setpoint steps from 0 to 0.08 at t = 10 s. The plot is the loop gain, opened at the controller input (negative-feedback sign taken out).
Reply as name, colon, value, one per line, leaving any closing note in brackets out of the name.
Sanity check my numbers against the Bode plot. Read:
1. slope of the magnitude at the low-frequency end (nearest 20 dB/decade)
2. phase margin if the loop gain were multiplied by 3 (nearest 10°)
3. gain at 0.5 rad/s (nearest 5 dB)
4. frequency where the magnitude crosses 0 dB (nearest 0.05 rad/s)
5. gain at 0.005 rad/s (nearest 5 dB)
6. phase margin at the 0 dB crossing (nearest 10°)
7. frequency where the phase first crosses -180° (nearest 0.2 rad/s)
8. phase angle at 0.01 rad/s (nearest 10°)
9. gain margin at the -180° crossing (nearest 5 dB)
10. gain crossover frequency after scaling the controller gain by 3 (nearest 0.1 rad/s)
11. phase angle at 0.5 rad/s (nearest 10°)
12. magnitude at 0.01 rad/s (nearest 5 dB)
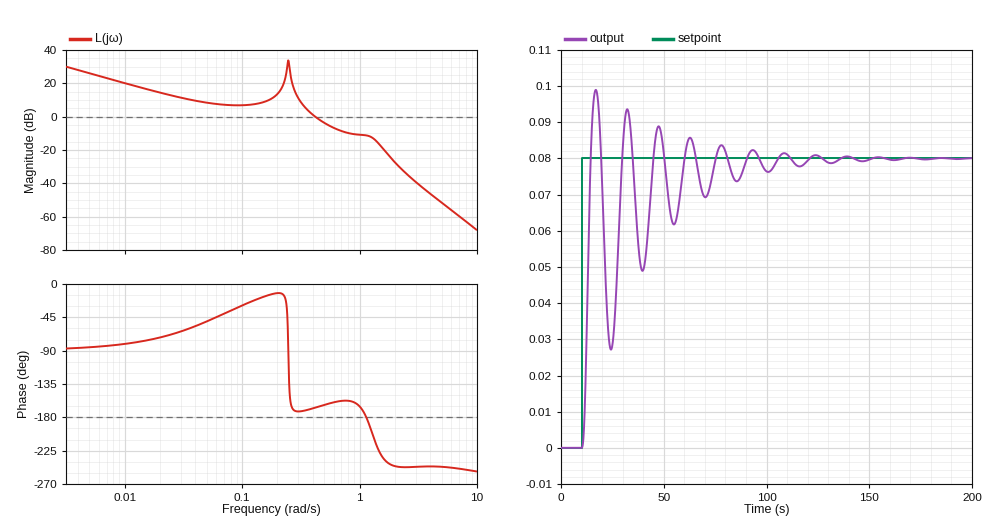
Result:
slope of the magnitude at the low-frequency end: -20 dB/decade
phase margin if the loop gain were multiplied by 3: 20°
gain at 0.5 rad/s: -5 dB
frequency where the magnitude crosses 0 dB: 0.40 rad/s
gain at 0.005 rad/s: 25 dB
phase margin at the 0 dB crossing: 10°
frequency where the phase first crosses -180°: 1.2 rad/s
phase angle at 0.01 rad/s: -80°
gain margin at the -180° crossing: 10 dB
gain crossover frequency after scaling the controller gain by 3: 0.8 rad/s
phase angle at 0.5 rad/s: -160°
magnitude at 0.01 rad/s: 20 dB
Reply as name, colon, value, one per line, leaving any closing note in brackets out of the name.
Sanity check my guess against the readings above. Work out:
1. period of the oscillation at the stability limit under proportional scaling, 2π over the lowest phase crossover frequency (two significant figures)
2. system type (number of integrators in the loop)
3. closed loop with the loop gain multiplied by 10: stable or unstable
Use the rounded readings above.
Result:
period of the oscillation at the stability limit under proportional scaling, 2π over the lowest phase crossover frequency: 5.2 s
system type: 1
closed loop with the loop gain multiplied by 10: stable or unstable: unstable
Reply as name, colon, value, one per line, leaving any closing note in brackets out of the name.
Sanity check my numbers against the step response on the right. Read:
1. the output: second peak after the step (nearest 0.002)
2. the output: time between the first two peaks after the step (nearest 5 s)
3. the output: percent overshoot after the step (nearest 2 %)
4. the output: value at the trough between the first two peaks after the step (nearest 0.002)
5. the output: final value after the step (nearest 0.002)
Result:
the output: second peak after the step: 0.094
the output: time between the first two peaks after the step: 15 s
the output: percent overshoot after the step: 24 %
the output: value at the trough between the first two peaks after the step: 0.028
the output: final value after the step: 0.080
